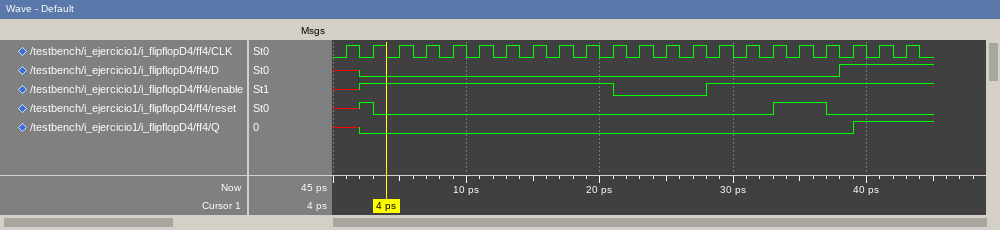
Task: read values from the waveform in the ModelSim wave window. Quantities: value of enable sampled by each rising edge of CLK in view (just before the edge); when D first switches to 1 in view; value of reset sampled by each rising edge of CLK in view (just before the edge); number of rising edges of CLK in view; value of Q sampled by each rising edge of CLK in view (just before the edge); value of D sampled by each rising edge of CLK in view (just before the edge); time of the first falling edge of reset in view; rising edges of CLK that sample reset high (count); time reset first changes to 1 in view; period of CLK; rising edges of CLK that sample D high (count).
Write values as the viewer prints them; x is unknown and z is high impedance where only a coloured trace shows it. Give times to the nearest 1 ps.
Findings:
x 1 1 1 1 1 1 1 1 1 1 0 0 0 1 1 1 1 1 1 1 1
38 ps
x 1 0 0 0 0 0 0 0 0 0 0 0 0 0 0 0 1 1 0 0 0
22
x 0 0 0 0 0 0 0 0 0 0 0 0 0 0 0 0 0 0 0 1 1
x 0 0 0 0 0 0 0 0 0 0 0 0 0 0 0 0 0 0 1 1 1
3 ps
3
2 ps
2 ps
3
